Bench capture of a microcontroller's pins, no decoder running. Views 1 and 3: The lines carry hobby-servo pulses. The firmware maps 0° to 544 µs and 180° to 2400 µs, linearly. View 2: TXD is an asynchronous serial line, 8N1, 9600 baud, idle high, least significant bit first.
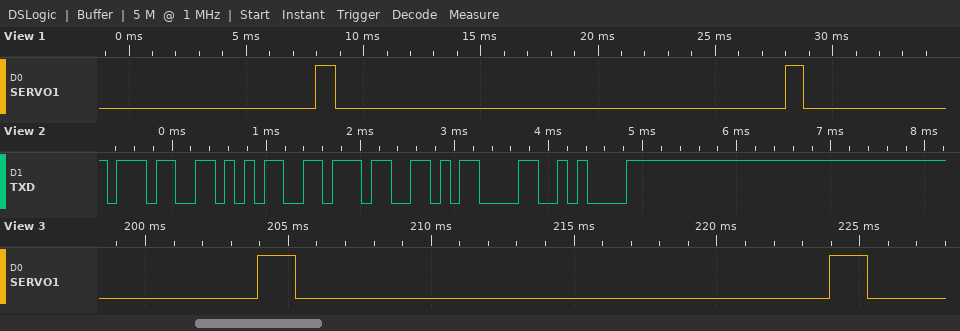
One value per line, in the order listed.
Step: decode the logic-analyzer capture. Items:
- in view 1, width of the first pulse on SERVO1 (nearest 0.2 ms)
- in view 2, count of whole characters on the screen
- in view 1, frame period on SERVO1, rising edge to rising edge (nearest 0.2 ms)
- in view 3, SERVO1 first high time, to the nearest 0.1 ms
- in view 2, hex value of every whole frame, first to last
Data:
0.8 ms
5
20.0 ms
1.3 ms
37 35 37 0D 0A
